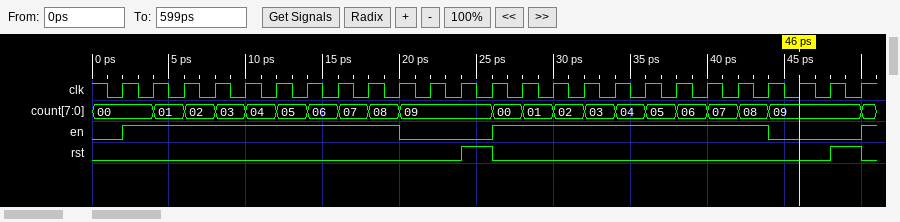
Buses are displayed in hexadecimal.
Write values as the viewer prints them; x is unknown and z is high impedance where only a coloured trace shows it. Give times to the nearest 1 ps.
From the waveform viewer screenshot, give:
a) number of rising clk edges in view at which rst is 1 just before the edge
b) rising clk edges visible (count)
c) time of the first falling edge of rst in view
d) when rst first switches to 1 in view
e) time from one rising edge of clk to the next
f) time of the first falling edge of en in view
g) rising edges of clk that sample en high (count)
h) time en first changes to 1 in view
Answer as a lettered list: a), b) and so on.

a) 2
b) 25
c) 26 ps
d) 24 ps
e) 2 ps
f) 20 ps
g) 18
h) 2 ps
